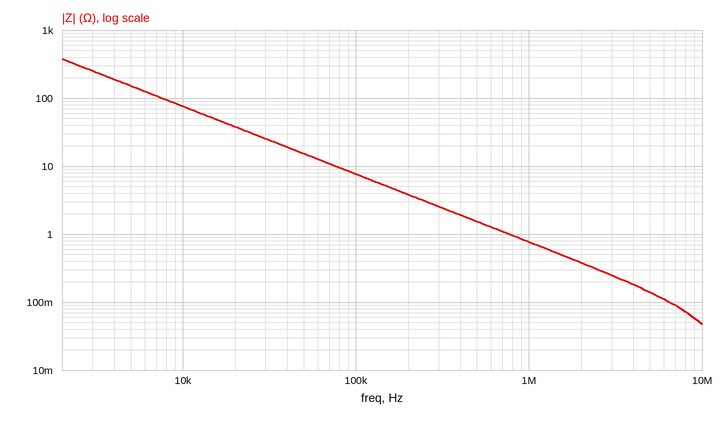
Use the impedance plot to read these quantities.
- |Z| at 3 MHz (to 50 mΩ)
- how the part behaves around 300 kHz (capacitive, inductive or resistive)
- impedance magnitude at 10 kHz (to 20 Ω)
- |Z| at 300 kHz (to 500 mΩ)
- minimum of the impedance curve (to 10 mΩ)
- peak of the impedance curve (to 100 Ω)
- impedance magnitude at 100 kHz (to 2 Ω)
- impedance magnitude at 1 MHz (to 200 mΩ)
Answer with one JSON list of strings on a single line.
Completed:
["250 mΩ", "capacitive", "80 Ω", "2.5 Ω", "50 mΩ", "400 Ω", "8 Ω", "800 mΩ"]
